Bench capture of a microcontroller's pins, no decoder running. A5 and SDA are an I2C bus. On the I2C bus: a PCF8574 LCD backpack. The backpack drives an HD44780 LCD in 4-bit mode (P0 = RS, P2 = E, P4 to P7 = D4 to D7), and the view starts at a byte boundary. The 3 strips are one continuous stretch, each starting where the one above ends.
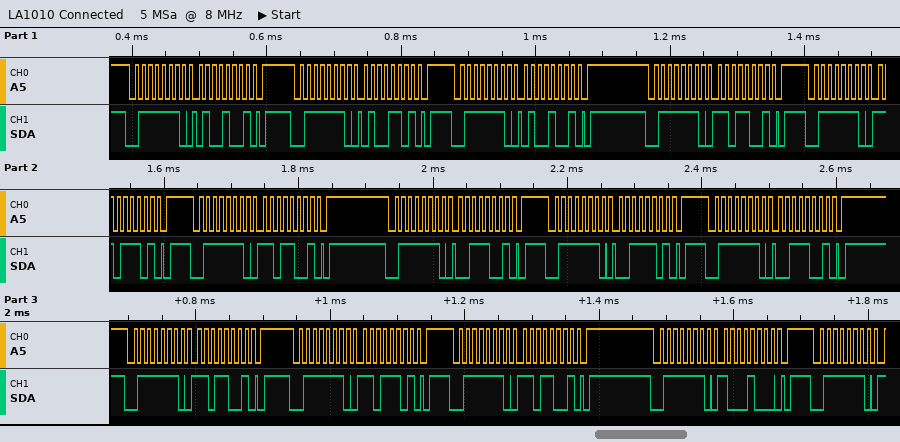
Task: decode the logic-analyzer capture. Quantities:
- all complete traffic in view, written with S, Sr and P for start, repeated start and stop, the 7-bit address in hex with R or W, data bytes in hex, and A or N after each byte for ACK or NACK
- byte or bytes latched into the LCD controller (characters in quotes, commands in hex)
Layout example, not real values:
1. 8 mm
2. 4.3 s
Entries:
1. S 3FW A 49 A P S 3FW A 4D A P S 3FW A 49 A P S 3FW A D9 A P S 3FW A DD A P S 3FW A D9 A P S 3FW A 39 A P S 3FW A 3D A P S 3FW A 39 A P S 3FW A D9 A P S 3FW A DD A P S 3FW A D9 A P S 3FW A 88 A P S 3FW A
2. 'M' '='
